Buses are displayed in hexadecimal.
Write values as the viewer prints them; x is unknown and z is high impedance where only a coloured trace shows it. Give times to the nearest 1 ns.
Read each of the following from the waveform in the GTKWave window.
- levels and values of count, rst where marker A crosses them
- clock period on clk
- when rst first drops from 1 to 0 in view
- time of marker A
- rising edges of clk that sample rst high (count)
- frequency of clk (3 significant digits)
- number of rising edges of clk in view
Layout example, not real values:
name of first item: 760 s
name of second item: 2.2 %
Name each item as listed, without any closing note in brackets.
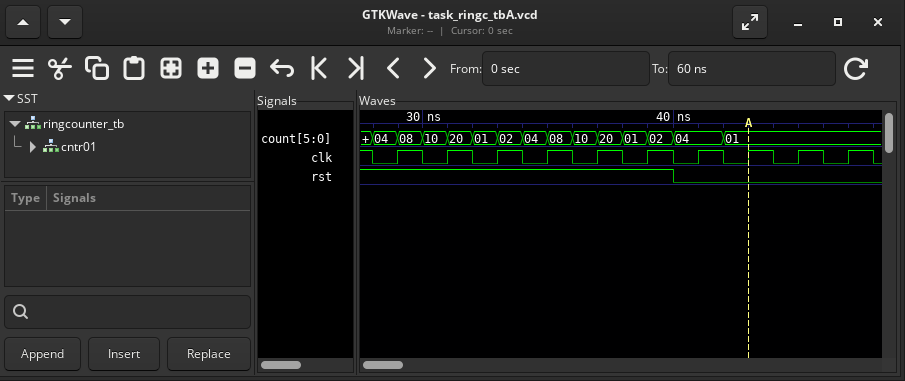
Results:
levels and values of count, rst where marker A crosses them: count=01, rst=0
clock period on clk: 2 ns
when rst first drops from 1 to 0 in view: 40 ns
time of marker A: 43 ns
rising edges of clk that sample rst high: 6
frequency of clk: 500 MHz
number of rising edges of clk in view: 10
